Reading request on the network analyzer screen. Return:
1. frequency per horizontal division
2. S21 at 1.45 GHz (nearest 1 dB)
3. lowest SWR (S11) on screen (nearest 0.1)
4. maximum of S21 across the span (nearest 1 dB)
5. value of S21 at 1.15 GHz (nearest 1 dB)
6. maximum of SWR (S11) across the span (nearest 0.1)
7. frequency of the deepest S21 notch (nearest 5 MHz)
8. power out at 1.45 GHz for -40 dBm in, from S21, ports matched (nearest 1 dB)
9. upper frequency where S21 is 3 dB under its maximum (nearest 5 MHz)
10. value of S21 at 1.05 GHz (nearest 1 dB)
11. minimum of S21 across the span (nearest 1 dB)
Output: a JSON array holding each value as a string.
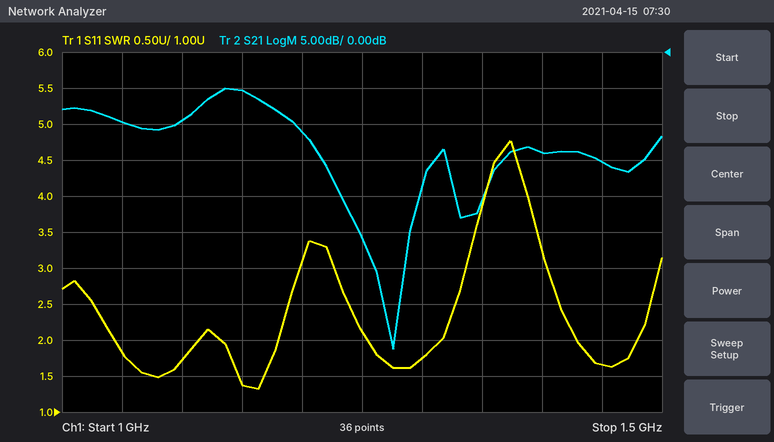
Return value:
["50 MHz", "-15 dB", "1.3", "-5 dB", "-5 dB", "4.8", "1.275 GHz", "-55 dBm", "1.180 GHz", "-10 dB", "-41 dB"]
